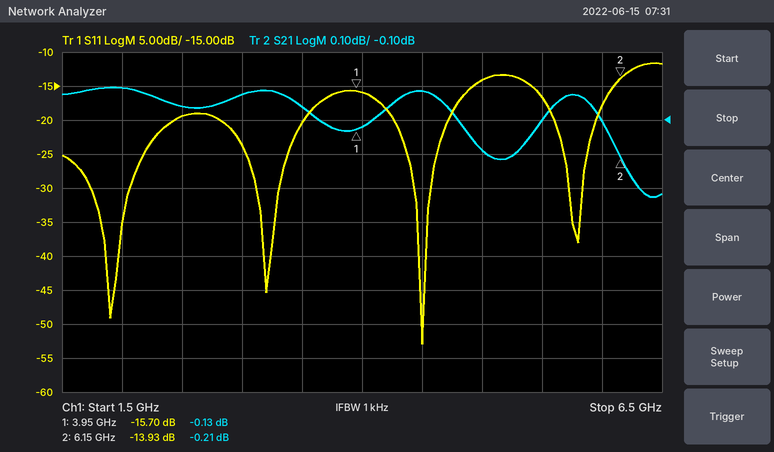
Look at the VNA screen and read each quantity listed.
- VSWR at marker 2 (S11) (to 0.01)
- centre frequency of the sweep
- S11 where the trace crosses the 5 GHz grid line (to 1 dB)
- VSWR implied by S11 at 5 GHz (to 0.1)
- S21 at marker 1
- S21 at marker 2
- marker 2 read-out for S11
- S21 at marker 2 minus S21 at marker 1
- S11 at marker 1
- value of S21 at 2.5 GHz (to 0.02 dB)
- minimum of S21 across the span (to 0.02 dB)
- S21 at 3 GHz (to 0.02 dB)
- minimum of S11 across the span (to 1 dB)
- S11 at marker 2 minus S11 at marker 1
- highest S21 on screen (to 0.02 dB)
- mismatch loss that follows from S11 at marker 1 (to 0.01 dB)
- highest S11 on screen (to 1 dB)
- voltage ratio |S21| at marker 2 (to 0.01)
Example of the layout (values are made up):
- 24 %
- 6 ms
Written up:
- 1.50
- 4 GHz
- -14 dB
- 1.5
- -0.13 dB
- -0.21 dB
- -13.93 dB
- -0.08 dB
- -15.70 dB
- -0.06 dB
- -0.32 dB
- -0.02 dB
- -53 dB
- 1.77 dB
- 0.00 dB
- 0.12 dB
- -12 dB
- 0.98
